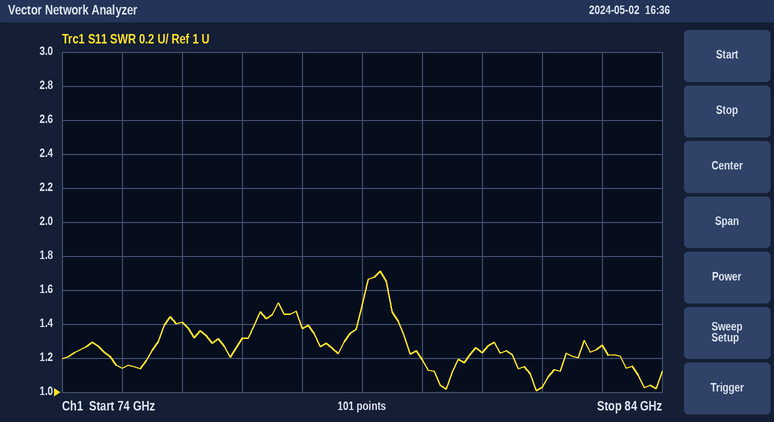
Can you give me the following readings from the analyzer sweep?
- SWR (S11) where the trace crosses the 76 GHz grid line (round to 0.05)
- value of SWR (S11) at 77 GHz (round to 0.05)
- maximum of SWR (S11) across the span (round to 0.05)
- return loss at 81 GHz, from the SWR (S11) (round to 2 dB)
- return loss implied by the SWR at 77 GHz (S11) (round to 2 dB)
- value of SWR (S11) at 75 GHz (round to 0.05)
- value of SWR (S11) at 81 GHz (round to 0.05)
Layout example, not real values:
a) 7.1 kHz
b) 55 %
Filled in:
a) 1.40
b) 1.30
c) 1.70
d) 20 dB
e) 18 dB
f) 1.15
g) 1.25
